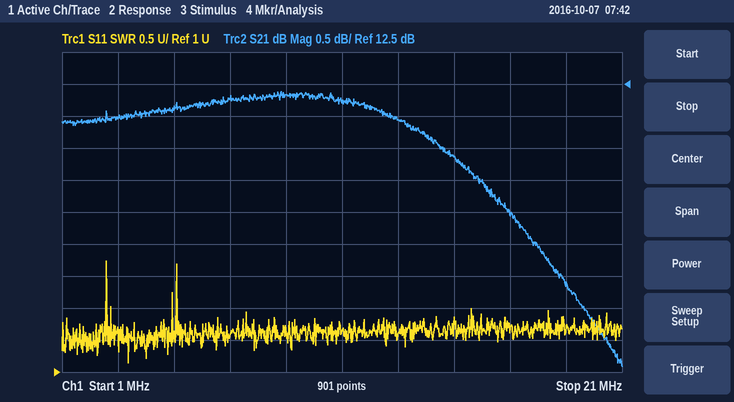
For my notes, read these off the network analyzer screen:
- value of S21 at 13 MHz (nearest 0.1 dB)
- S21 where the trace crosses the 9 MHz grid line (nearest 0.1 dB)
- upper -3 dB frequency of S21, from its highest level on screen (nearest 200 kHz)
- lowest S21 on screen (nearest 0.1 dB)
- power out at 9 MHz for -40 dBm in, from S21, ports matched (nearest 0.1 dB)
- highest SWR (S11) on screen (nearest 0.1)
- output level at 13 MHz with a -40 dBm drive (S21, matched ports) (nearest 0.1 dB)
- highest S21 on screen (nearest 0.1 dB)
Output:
11.9 dB
12.3 dB
19.0 MHz
8.1 dB
-27.7 dBm
2.7
-28.1 dBm
12.4 dB
